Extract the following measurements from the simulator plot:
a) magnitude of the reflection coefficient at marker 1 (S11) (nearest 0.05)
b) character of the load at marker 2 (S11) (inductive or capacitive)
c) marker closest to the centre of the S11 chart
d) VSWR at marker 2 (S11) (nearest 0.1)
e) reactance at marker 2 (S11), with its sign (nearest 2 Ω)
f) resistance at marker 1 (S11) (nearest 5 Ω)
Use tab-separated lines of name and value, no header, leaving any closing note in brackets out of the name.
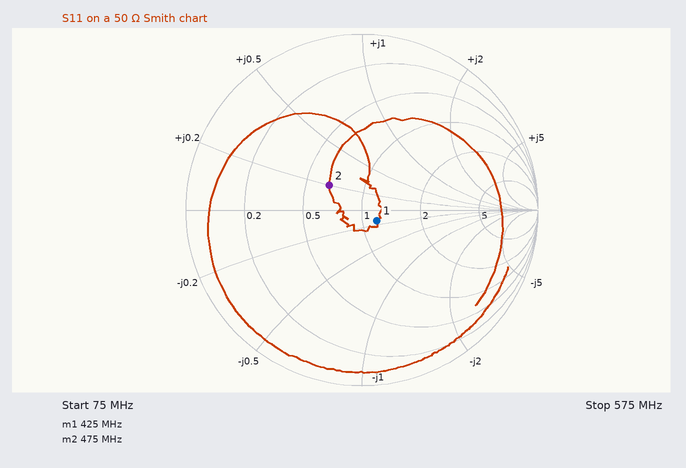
magnitude of the reflection coefficient at marker 1 (S11)	0.10
character of the load at marker 2 (S11)	inductive
marker closest to the centre of the S11 chart	marker 1
VSWR at marker 2 (S11)	1.6
reactance at marker 2 (S11), with its sign	+10 Ω
resistance at marker 1 (S11)	60 Ω
